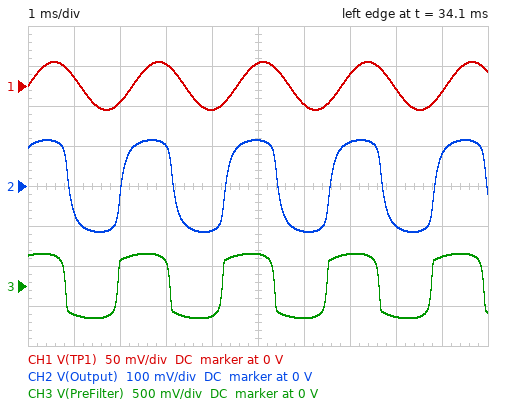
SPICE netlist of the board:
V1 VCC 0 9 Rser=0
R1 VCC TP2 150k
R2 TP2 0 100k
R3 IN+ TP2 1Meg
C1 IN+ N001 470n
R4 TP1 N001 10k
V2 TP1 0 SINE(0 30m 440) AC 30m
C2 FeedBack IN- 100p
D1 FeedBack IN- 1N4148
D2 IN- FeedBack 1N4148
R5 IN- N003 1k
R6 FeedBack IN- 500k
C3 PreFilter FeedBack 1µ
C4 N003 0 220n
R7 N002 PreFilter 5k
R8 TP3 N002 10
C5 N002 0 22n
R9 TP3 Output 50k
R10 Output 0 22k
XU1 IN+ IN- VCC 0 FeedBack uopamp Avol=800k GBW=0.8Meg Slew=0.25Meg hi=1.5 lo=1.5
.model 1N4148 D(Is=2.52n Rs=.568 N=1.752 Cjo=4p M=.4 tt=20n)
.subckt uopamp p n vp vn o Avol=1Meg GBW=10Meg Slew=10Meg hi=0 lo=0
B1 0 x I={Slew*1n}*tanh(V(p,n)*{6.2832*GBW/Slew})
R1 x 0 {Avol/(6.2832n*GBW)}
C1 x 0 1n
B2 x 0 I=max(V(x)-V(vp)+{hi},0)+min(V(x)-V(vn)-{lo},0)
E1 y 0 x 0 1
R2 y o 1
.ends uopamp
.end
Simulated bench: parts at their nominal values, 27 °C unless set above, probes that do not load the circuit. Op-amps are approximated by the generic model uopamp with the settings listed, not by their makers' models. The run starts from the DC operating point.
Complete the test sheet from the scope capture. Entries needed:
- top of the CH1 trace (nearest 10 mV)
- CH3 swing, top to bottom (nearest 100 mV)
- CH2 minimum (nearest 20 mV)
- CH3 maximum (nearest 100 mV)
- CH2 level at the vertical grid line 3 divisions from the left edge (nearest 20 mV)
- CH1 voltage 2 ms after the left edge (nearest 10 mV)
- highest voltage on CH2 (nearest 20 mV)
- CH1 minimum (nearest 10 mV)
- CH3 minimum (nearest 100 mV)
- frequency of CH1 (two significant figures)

30 mV
800 mV
-120 mV
400 mV
100 mV
-20 mV
120 mV
-30 mV
-400 mV
440 Hz
